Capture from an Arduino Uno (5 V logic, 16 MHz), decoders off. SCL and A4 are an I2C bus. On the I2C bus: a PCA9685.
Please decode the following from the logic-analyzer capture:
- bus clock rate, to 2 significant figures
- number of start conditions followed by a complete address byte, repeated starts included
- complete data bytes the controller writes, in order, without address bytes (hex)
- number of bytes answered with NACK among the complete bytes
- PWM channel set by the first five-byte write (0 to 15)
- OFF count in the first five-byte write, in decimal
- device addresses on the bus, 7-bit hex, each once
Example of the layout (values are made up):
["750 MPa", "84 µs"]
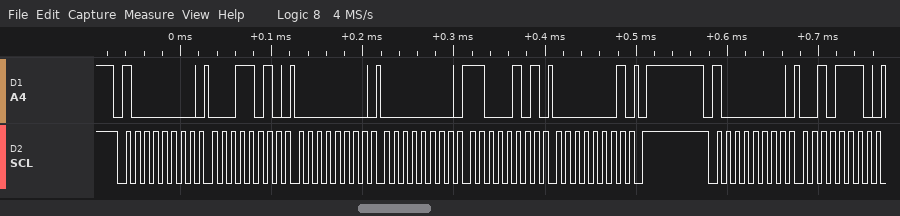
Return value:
["100 kHz", "2", "1A 00 00 C5 01 2E", "0", "5", "453", "0x40"]
